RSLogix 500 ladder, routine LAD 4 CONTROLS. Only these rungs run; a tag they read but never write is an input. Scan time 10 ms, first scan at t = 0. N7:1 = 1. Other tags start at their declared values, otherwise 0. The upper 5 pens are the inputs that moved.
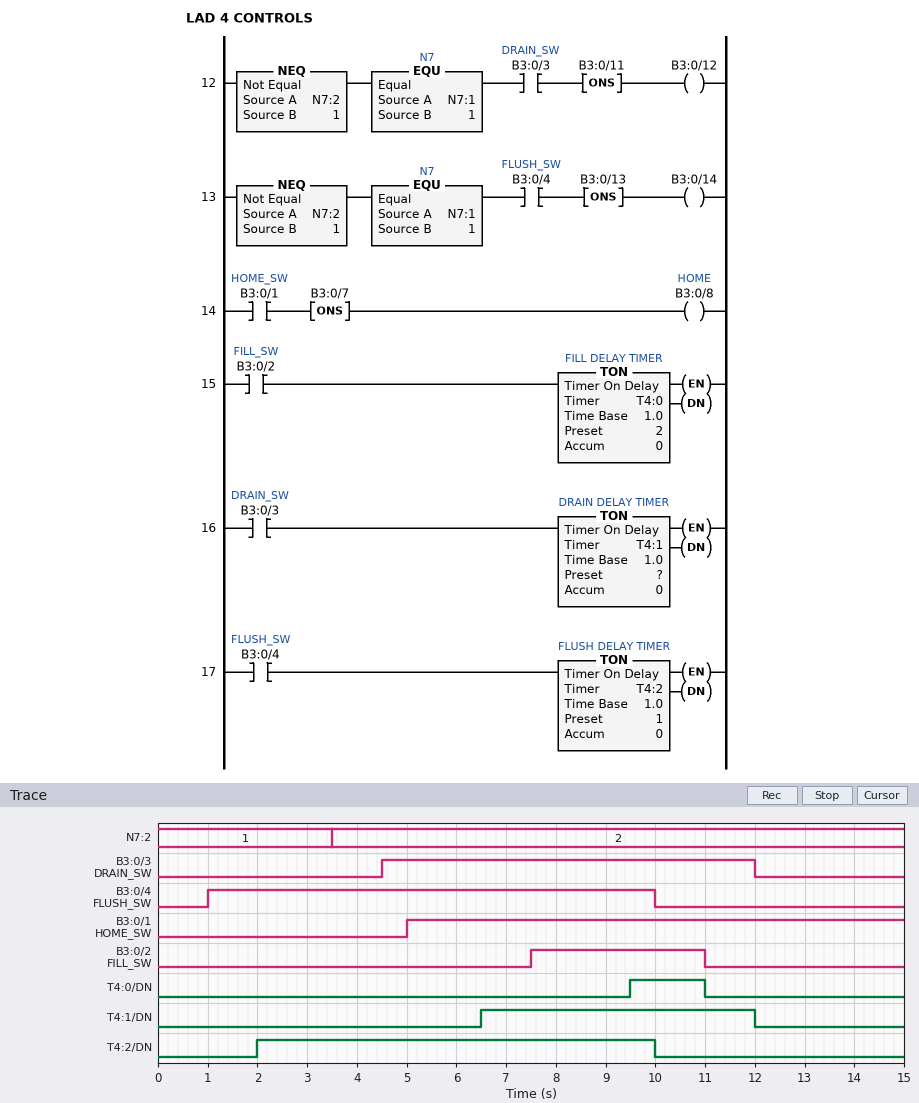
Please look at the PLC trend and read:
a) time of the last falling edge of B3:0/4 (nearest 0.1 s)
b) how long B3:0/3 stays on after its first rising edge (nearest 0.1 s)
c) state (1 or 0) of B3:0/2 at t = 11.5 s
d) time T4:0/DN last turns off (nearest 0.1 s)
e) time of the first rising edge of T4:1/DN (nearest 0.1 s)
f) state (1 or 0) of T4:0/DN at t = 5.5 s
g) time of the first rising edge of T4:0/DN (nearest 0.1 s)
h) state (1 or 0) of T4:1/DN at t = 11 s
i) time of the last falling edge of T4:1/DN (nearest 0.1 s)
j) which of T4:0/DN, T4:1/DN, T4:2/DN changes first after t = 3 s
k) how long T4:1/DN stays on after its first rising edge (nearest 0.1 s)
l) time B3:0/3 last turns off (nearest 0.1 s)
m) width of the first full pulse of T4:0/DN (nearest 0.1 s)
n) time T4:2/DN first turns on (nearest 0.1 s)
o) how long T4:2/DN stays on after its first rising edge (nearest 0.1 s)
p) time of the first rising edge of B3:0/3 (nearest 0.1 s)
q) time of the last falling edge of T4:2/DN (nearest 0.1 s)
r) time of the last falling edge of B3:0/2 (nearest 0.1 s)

10.0 s
7.5 s
0
11.0 s
6.5 s
0
9.5 s
1
12.0 s
T4:1/DN
5.5 s
12.0 s
1.5 s
2.0 s
8.0 s
4.5 s
10.0 s
11.0 s
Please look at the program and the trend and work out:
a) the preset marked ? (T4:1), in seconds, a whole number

2 s
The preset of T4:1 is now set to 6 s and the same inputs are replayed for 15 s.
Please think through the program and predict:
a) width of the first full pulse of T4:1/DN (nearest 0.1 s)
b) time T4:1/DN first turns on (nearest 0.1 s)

1.5 s
10.5 s
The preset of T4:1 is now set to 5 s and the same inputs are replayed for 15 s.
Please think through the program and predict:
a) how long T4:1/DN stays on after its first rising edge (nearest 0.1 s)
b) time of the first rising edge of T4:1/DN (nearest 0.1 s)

2.5 s
9.5 s
